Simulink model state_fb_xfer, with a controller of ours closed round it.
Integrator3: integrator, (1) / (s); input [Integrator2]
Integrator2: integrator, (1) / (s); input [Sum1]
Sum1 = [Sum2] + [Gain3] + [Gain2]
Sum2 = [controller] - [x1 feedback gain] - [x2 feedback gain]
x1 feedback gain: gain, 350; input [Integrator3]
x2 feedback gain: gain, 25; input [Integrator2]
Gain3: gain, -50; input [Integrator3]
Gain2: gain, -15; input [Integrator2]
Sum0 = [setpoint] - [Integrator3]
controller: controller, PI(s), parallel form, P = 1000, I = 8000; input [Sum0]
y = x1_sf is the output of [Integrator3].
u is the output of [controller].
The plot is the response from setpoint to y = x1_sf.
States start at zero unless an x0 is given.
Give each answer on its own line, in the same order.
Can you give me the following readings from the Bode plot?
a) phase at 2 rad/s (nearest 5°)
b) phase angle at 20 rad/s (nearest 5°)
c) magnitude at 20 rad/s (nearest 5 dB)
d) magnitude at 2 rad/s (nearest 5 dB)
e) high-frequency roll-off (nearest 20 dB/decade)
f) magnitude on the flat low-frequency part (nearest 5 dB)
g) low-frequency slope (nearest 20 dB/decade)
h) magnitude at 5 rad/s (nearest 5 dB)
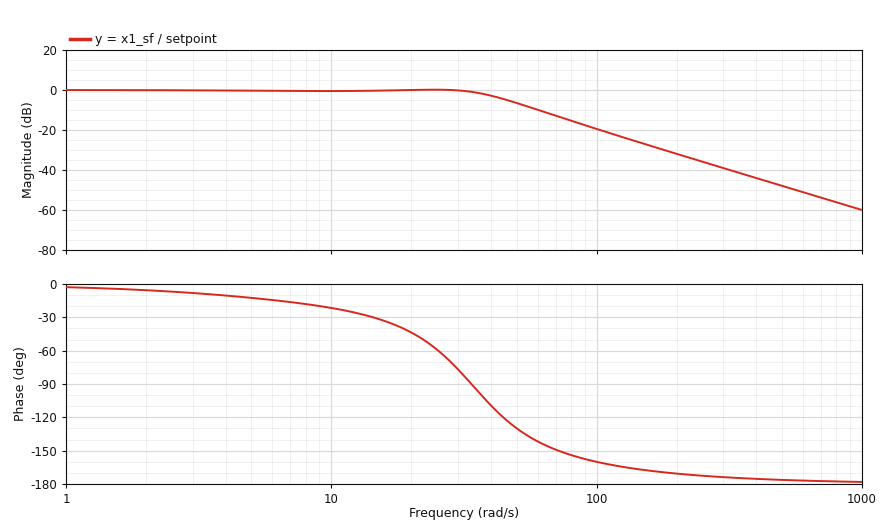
-5°
-45°
0 dB
0 dB
-40 dB/decade
0 dB
0 dB/decade
0 dB
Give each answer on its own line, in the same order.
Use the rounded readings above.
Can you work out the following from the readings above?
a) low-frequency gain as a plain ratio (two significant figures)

1.0
